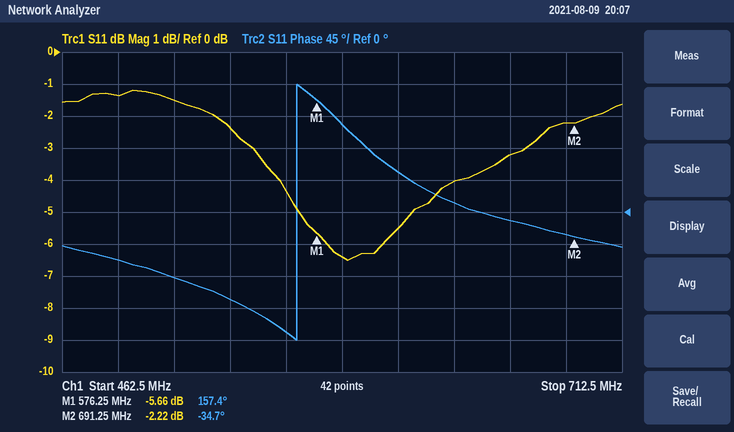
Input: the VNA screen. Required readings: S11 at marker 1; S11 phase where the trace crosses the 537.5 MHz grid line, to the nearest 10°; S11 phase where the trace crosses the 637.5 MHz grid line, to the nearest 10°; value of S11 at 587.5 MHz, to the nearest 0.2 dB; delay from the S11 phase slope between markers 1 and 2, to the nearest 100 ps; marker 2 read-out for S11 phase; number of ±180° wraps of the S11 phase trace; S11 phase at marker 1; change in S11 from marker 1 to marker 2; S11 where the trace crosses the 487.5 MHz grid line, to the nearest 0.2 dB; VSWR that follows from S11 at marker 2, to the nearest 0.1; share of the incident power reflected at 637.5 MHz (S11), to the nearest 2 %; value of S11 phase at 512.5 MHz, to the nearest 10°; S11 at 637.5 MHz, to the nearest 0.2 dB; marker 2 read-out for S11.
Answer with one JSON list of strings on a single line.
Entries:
["-5.66 dB", "-120°", "10°", "-6.4 dB", "4.6 ns", "-34.7°", "1", "157.4°", "3.44 dB", "-1.4 dB", "7.9", "40 %", "-90°", "-4.0 dB", "-2.22 dB"]
